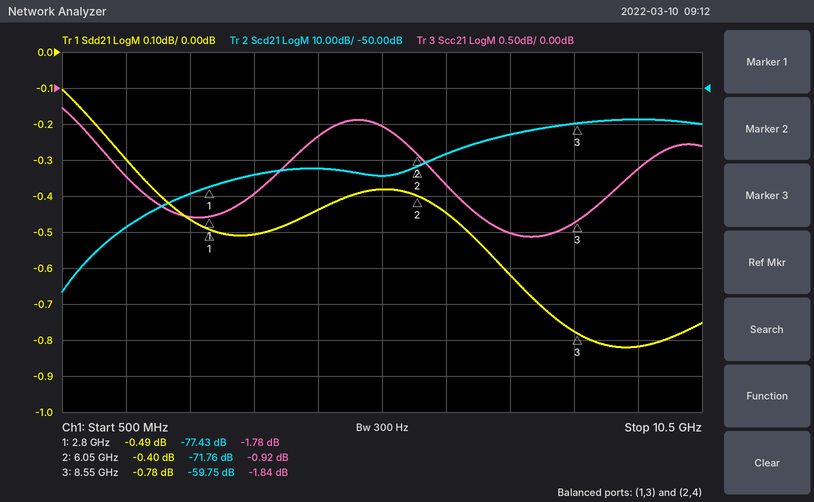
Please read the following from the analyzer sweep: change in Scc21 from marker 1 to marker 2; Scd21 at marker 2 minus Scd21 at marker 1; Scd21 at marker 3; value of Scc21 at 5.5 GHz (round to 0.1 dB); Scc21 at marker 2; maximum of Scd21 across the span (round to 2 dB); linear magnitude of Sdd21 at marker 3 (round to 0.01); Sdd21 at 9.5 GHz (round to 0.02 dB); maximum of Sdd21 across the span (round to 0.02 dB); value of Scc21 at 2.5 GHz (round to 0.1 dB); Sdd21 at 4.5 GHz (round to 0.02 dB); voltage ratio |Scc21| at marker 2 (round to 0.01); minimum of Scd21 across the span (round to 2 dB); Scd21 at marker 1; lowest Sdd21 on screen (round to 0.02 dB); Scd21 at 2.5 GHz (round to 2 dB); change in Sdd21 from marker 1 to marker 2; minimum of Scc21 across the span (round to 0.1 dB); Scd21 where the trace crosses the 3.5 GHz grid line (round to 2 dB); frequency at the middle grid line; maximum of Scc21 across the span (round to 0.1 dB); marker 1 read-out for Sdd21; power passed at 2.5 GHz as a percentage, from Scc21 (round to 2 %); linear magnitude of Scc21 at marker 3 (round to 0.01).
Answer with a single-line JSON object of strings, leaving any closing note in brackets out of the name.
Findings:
{"change in Scc21 from marker 1 to marker 2": "0.86 dB", "Scd21 at marker 2 minus Scd21 at marker 1": "5.67 dB", "Scd21 at marker 3": "-59.75 dB", "value of Scc21 at 5.5 GHz": "-0.5 dB", "Scc21 at marker 2": "-0.92 dB", "maximum of Scd21 across the span": "-58 dB", "linear magnitude of Sdd21 at marker 3": "0.91", "Sdd21 at 9.5 GHz": "-0.82 dB", "maximum of Sdd21 across the span": "-0.10 dB", "value of Scc21 at 2.5 GHz": "-1.8 dB", "Sdd21 at 4.5 GHz": "-0.44 dB", "voltage ratio |Scc21| at marker 2": "0.90", "minimum of Scd21 across the span": "-106 dB", "Scd21 at marker 1": "-77.43 dB", "lowest Sdd21 on screen": "-0.82 dB", "Scd21 at 2.5 GHz": "-80 dB", "change in Sdd21 from marker 1 to marker 2": "0.09 dB", "minimum of Scc21 across the span": "-2.1 dB", "Scd21 where the trace crosses the 3.5 GHz grid line": "-74 dB", "frequency at the middle grid line": "5.5 GHz", "maximum of Scc21 across the span": "-0.3 dB", "marker 1 read-out for Sdd21": "-0.49 dB", "power passed at 2.5 GHz as a percentage, from Scc21": "66 %", "linear magnitude of Scc21 at marker 3": "0.81"}
